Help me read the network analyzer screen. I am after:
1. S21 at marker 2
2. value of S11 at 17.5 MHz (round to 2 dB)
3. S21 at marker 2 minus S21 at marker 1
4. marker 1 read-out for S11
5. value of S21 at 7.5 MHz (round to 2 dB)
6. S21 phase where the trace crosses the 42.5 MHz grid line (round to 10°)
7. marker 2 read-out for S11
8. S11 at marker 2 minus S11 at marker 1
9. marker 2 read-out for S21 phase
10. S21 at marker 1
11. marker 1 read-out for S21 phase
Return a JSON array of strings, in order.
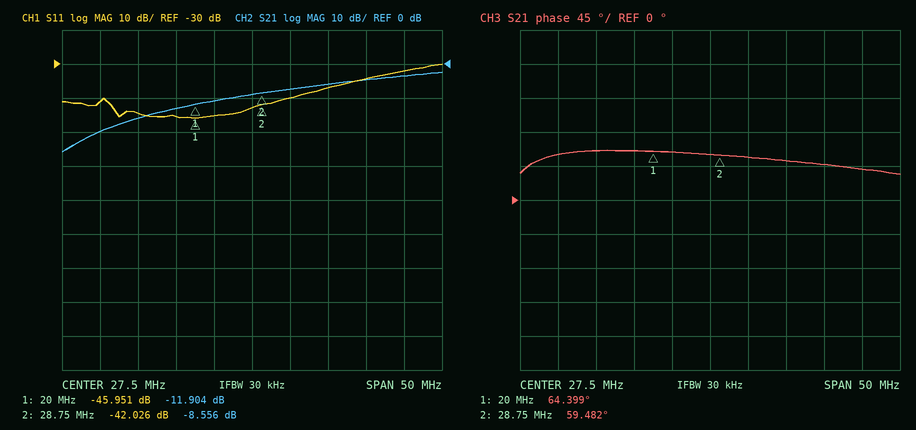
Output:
["-8.556 dB", "-46 dB", "3.348 dB", "-45.951 dB", "-20 dB", "50°", "-42.026 dB", "3.925 dB", "59.482°", "-11.904 dB", "64.399°"]
